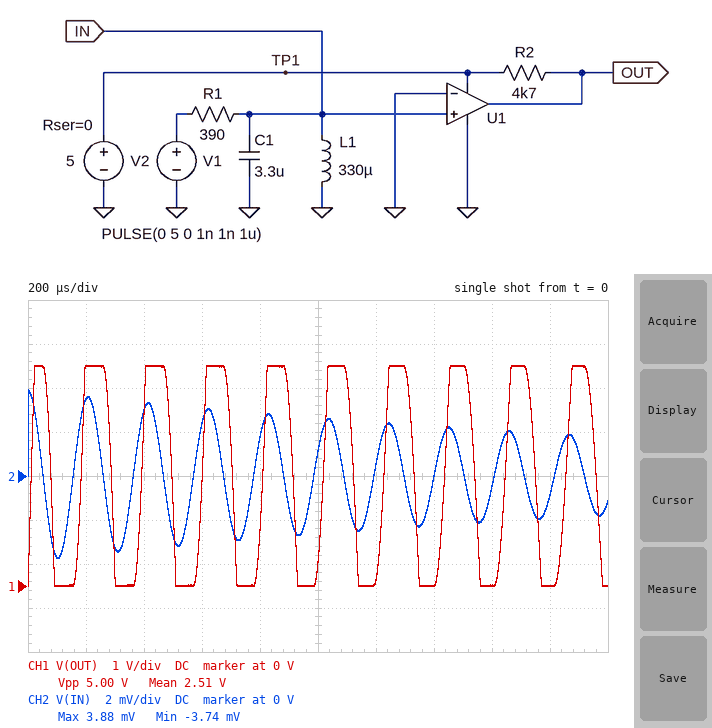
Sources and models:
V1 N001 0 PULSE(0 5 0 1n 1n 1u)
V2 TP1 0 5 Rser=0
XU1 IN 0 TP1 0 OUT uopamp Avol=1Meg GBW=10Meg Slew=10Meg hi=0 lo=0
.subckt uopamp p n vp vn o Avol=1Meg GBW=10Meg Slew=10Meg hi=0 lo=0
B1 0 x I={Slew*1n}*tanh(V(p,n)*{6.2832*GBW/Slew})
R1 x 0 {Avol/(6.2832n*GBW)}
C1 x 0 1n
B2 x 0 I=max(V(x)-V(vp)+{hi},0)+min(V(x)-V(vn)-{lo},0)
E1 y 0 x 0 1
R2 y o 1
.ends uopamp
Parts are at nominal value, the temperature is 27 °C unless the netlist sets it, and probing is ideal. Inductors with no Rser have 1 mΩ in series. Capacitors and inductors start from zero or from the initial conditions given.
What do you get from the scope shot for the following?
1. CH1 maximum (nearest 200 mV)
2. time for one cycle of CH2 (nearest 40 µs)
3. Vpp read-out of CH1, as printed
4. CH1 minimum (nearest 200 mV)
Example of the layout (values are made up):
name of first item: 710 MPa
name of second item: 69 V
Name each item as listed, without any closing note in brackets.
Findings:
CH1 maximum: 5.0 V
time for one cycle of CH2: 200 µs
Vpp read-out of CH1, as printed: 5.00 V
CH1 minimum: 0 V
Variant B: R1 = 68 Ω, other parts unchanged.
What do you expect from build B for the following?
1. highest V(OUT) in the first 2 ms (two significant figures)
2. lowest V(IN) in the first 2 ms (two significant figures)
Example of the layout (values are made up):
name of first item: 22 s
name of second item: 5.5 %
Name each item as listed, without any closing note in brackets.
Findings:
highest V(OUT) in the first 2 ms: 5.0 V
lowest V(IN) in the first 2 ms: -18 mV
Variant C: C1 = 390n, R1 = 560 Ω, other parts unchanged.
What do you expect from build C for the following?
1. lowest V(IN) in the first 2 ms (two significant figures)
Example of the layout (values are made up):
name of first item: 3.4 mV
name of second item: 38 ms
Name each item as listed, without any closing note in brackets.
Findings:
lowest V(IN) in the first 2 ms: -21 mV
